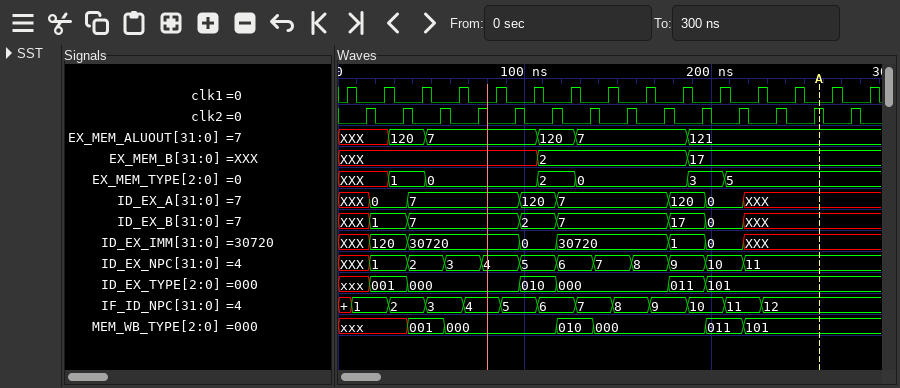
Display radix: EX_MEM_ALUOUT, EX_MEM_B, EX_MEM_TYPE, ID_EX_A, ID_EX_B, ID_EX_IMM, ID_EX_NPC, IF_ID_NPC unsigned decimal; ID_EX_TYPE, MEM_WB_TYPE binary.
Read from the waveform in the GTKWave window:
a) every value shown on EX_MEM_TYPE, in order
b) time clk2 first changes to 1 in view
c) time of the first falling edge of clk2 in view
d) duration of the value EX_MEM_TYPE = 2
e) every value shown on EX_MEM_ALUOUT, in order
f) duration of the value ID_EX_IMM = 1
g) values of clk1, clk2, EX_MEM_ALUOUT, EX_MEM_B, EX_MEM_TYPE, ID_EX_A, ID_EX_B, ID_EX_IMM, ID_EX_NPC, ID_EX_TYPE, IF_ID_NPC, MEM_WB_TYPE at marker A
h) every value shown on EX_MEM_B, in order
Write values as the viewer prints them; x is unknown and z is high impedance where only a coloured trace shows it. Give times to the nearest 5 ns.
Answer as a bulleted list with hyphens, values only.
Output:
- XXX, 1, 0, 2, 0, 3, 5
- 15 ns
- 20 ns
- 20 ns
- XXX, 120, 7, 120, 7, 121
- 20 ns
- clk1=0, clk2=1, EX_MEM_ALUOUT=121, EX_MEM_B=17, EX_MEM_TYPE=5, ID_EX_A=XXX, ID_EX_B=XXX, ID_EX_IMM=XXX, ID_EX_NPC=11, ID_EX_TYPE=101, IF_ID_NPC=12, MEM_WB_TYPE=101
- XXX, 2, 17
